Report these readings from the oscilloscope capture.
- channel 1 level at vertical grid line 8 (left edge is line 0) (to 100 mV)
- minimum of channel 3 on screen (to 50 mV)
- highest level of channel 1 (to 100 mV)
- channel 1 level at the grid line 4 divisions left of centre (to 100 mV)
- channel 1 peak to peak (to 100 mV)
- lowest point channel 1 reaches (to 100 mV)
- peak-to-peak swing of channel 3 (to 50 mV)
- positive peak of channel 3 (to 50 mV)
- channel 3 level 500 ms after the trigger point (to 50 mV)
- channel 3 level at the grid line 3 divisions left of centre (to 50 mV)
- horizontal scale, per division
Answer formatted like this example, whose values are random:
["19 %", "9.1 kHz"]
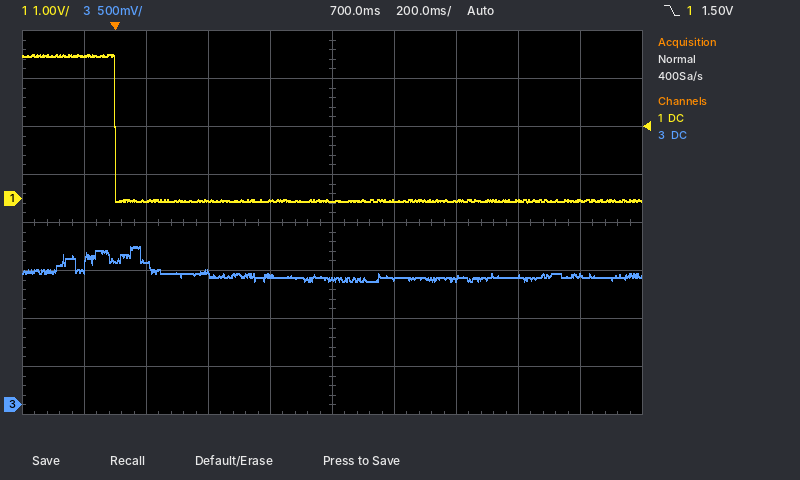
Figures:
["0.0 V", "1.30 V", "3.0 V", "3.0 V", "3.1 V", "-100 mV", "350 mV", "1.65 V", "1.35 V", "1.50 V", "200 ms"]
